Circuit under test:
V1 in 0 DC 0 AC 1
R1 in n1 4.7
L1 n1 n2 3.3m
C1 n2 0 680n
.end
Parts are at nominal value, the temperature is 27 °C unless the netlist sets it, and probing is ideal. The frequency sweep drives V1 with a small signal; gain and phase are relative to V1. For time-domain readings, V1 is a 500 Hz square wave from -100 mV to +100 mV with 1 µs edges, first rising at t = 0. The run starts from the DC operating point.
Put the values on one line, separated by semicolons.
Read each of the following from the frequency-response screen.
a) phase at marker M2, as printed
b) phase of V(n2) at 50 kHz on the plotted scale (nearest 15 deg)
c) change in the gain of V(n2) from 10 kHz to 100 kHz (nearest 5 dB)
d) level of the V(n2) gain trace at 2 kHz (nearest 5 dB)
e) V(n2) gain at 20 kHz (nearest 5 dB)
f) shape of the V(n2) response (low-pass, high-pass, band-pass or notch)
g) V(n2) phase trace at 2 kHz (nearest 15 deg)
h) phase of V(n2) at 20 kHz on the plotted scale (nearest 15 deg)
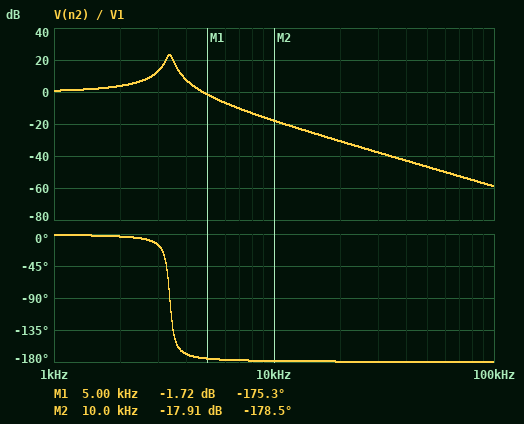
-178.5 deg; -180 deg; -40 dB; 5 dB; -30 dB; low-pass; 0 deg; -180 deg
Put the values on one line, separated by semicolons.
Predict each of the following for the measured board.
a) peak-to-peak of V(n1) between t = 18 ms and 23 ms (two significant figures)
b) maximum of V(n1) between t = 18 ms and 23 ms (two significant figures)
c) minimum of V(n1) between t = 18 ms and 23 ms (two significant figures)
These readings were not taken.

230 mV; 110 mV; -110 mV
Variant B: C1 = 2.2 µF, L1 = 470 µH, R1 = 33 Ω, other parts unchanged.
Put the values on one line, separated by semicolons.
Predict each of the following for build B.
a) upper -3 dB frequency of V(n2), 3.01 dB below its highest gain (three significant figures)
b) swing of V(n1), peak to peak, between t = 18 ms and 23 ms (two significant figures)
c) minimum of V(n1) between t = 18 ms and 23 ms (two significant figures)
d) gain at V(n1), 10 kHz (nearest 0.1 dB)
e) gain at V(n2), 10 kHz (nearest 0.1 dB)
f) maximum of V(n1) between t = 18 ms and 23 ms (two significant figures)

2.69 kHz; 200 mV; -100 mV; -5.0 dB; -14.8 dB; 100 mV
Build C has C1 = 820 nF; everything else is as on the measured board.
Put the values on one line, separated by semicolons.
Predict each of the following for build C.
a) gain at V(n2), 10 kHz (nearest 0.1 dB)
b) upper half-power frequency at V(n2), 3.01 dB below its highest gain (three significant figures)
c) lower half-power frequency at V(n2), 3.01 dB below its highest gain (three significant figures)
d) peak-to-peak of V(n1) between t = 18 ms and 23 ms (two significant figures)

-19.7 dB; 3.17 kHz; 2.94 kHz; 220 mV
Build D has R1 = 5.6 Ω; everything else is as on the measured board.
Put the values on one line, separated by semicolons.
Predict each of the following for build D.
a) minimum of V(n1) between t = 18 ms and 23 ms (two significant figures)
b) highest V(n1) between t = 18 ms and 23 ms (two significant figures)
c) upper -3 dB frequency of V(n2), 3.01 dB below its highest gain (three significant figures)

-120 mV; 120 mV; 3.49 kHz
